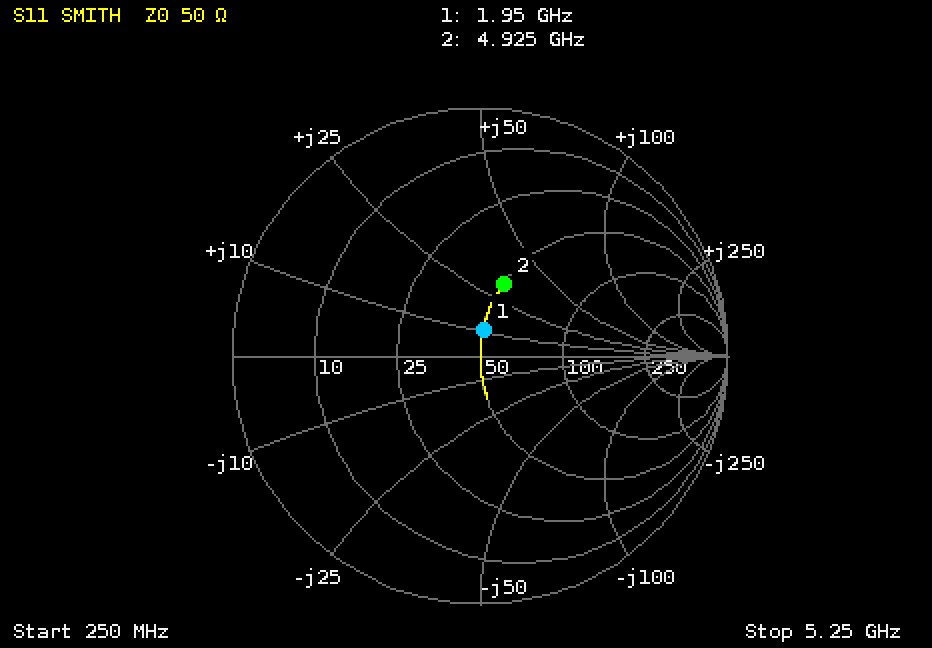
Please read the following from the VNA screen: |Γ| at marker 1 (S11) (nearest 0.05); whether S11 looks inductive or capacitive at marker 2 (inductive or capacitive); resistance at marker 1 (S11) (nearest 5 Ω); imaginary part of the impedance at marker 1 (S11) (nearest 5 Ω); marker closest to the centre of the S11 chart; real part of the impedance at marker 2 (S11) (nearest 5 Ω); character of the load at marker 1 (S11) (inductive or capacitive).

0.10
inductive
50 Ω
+10 Ω
marker 1
50 Ω
inductive
